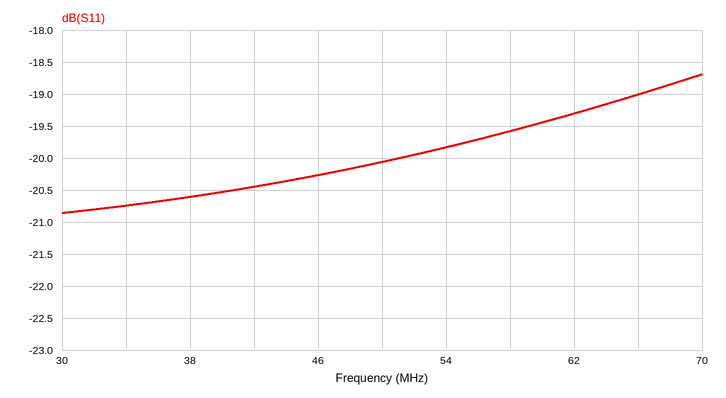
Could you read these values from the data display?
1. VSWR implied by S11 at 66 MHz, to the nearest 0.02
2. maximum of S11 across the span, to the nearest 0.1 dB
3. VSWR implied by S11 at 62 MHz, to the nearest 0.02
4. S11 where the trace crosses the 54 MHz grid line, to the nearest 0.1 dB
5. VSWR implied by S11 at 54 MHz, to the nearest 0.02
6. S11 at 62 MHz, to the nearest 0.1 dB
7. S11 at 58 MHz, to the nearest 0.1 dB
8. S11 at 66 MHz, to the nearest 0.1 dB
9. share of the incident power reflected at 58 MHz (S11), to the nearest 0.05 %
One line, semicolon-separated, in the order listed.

1.26; -18.7 dB; 1.24; -19.8 dB; 1.22; -19.3 dB; -19.6 dB; -19.0 dB; 1.10 %
